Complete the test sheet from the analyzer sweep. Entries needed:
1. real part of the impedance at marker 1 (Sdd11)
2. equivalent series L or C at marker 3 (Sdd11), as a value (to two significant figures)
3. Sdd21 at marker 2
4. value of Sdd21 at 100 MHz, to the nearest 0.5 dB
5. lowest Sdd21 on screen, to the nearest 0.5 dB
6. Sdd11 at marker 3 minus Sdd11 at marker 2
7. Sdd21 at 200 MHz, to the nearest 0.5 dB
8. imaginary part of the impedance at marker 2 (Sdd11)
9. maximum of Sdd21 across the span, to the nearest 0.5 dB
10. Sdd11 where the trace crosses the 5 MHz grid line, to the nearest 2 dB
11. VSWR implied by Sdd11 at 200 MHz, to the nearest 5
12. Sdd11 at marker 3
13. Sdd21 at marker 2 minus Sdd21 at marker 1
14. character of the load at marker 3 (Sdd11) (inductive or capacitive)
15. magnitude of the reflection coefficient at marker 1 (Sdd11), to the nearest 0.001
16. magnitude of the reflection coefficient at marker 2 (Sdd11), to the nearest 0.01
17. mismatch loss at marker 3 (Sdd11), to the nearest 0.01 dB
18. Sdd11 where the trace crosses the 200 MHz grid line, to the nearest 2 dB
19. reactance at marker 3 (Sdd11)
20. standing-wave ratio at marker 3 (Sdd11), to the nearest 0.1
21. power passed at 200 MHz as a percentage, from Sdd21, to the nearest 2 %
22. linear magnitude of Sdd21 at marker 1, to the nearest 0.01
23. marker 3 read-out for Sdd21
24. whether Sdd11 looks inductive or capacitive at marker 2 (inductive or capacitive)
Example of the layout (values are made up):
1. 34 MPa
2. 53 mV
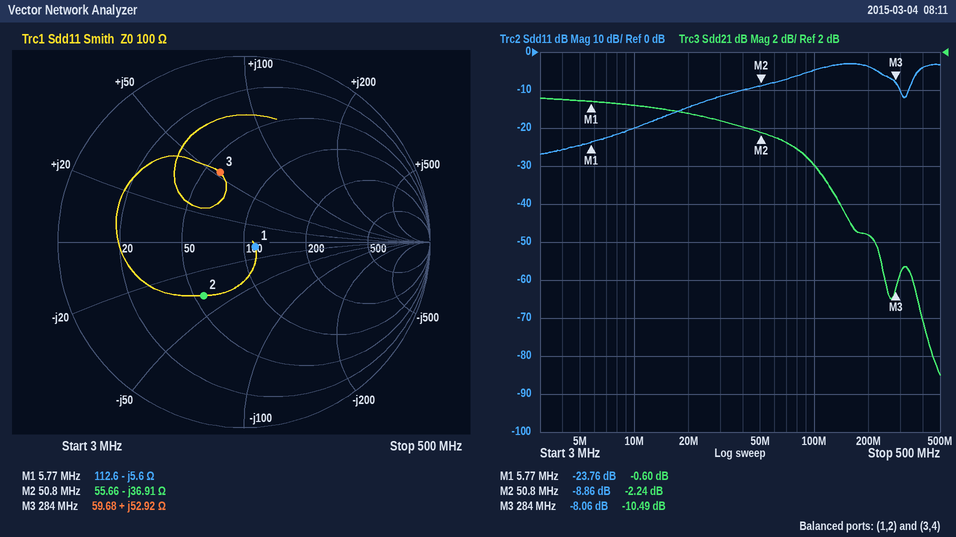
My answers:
1. 112.6 Ω
2. 30 nH
3. -2.24 dB
4. -4.0 dB
5. -15.0 dB
6. 0.80 dB
7. -7.5 dB
8. -36.91 Ω
9. -0.5 dB
10. -24 dB
11. 5
12. -8.06 dB
13. -1.64 dB
14. inductive
15. 0.065
16. 0.36
17. 0.74 dB
18. -4 dB
19. +52.92 Ω
20. 2.3
21. 18 %
22. 0.93
23. -10.49 dB
24. capacitive
